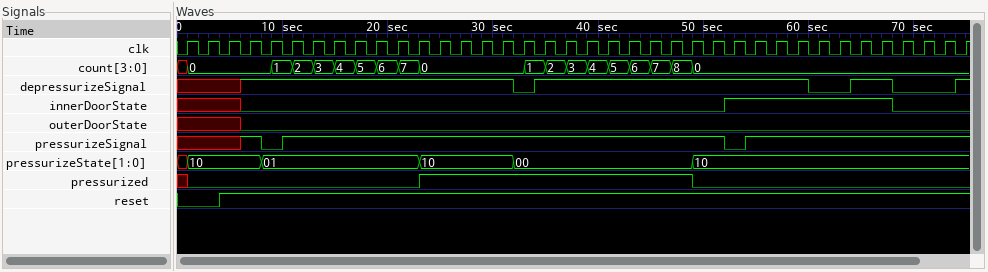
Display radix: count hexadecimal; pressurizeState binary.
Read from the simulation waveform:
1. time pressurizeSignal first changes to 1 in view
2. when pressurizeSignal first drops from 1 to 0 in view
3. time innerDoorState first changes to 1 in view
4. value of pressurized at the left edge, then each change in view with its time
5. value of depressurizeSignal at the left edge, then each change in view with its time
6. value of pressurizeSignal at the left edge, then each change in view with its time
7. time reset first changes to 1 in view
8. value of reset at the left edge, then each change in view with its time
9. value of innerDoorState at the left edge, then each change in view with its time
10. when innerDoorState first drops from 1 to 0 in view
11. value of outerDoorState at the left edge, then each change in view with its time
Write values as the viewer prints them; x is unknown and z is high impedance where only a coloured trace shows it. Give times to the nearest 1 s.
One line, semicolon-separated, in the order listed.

6 s; 8 s; 52 s; x, 0 at 1 s, 1 at 23 s, 0 at 49 s; x, 1 at 6 s, 0 at 32 s, 1 at 34 s, 0 at 60 s, 1 at 64 s, 0 at 68 s, 1 at 74 s; x, 1 at 6 s, 0 at 8 s, 1 at 10 s, 0 at 52 s, 1 at 54 s; 4 s; 0, 1 at 4 s; x, 0 at 6 s, 1 at 52 s, 0 at 68 s; 68 s; x, 0 at 6 s
